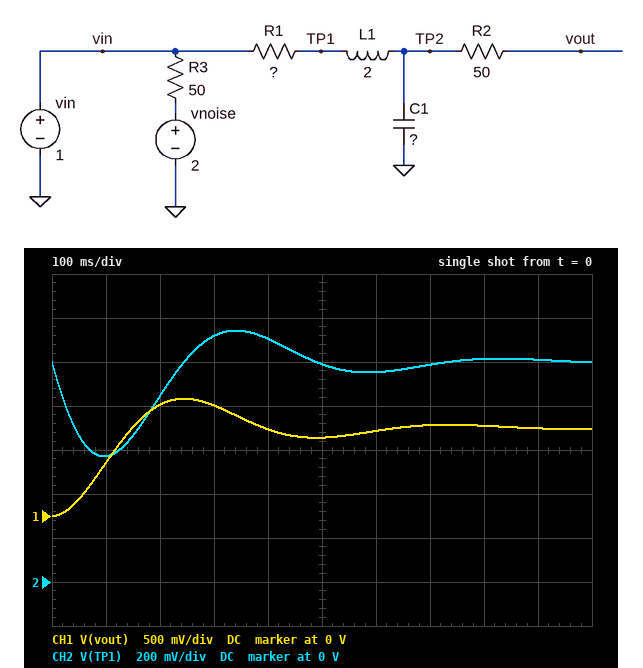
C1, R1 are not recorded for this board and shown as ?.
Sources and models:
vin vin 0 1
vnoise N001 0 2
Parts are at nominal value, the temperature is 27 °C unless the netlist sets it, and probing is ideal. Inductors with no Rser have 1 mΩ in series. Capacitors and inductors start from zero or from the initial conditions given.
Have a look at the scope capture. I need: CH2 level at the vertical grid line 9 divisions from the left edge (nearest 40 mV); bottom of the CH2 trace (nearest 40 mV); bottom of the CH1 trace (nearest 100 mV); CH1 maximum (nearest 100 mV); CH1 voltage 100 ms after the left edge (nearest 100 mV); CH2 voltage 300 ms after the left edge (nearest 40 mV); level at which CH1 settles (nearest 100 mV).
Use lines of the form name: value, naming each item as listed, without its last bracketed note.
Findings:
CH2 level at the vertical grid line 9 divisions from the left edge: 1.00 V
bottom of the CH2 trace: 560 mV
bottom of the CH1 trace: 0 V
CH1 maximum: 1.3 V
CH1 voltage 100 ms after the left edge: 600 mV
CH2 voltage 300 ms after the left edge: 1.12 V
level at which CH1 settles: 1.0 V
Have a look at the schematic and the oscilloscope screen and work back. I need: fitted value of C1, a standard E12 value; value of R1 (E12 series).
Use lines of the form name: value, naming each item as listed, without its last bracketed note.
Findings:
fitted value of C1, a standard E12 value: 2.7 mF
value of R1: 18 Ω
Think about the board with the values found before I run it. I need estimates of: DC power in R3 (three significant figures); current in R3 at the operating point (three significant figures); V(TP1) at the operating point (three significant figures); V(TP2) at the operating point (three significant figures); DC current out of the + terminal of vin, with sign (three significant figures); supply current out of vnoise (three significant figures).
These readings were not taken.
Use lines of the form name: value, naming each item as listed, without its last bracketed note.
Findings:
DC power in R3: 20.0 mW
current in R3 at the operating point: 20.0 mA
V(TP1) at the operating point: 1.00 V
V(TP2) at the operating point: 1.00 V
DC current out of the + terminal of vin, with sign: -20.0 mA
supply current out of vnoise: 20.0 mA
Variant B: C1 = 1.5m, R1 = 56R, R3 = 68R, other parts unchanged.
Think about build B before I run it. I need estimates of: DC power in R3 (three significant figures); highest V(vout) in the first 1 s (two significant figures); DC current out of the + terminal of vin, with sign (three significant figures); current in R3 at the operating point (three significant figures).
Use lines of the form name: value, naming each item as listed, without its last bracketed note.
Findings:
DC power in R3: 14.7 mW
highest V(vout) in the first 1 s: 1.0 V
DC current out of the + terminal of vin, with sign: -14.7 mA
current in R3 at the operating point: 14.7 mA
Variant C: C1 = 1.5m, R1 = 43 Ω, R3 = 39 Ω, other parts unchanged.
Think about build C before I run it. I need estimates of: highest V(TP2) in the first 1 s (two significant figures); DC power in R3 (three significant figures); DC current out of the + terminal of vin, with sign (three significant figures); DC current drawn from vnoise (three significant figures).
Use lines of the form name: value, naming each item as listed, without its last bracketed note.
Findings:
highest V(TP2) in the first 1 s: 1.1 V
DC power in R3: 25.6 mW
DC current out of the + terminal of vin, with sign: -25.6 mA
DC current drawn from vnoise: 25.6 mA
